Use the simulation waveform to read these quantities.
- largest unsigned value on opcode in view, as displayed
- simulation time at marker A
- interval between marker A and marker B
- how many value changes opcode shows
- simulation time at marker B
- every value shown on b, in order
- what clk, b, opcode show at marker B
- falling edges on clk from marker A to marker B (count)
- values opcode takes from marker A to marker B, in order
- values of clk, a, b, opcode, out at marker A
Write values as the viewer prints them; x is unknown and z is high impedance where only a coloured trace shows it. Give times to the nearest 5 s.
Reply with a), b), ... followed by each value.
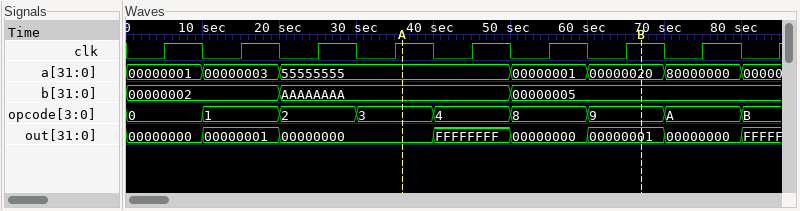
a) B
b) 35 s
c) 30 s
d) 8
e) 65 s
f) 00000002, AAAAAAAA, 00000005
g) clk=1, b=00000005, opcode=9
h) 3
i) 3, 4, 8, 9
j) clk=1, a=55555555, b=AAAAAAAA, opcode=3, out=00000000
